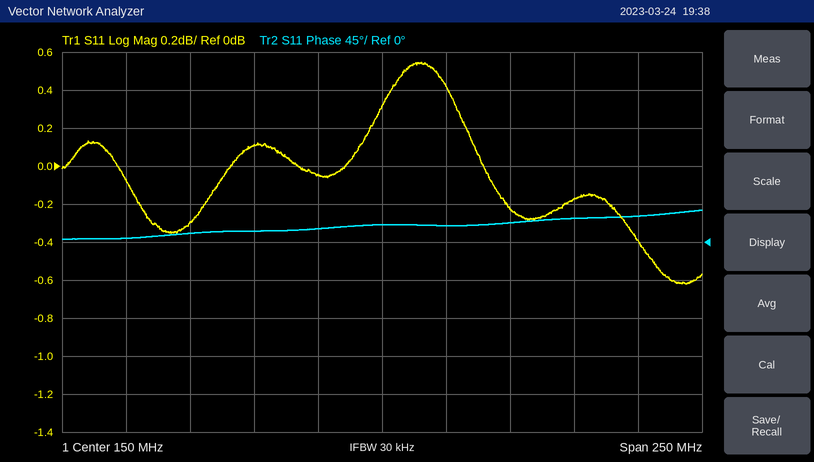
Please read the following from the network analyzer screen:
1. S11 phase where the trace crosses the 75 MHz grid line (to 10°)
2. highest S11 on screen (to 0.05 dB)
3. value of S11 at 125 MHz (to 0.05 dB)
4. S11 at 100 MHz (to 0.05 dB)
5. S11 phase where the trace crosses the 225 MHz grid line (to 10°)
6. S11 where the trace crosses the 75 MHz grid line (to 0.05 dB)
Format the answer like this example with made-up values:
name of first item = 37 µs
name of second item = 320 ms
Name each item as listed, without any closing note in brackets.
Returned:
S11 phase where the trace crosses the 75 MHz grid line = 10°
highest S11 on screen = 0.55 dB
value of S11 at 125 MHz = -0.05 dB
S11 at 100 MHz = 0.10 dB
S11 phase where the trace crosses the 225 MHz grid line = 30°
S11 where the trace crosses the 75 MHz grid line = -0.30 dB
